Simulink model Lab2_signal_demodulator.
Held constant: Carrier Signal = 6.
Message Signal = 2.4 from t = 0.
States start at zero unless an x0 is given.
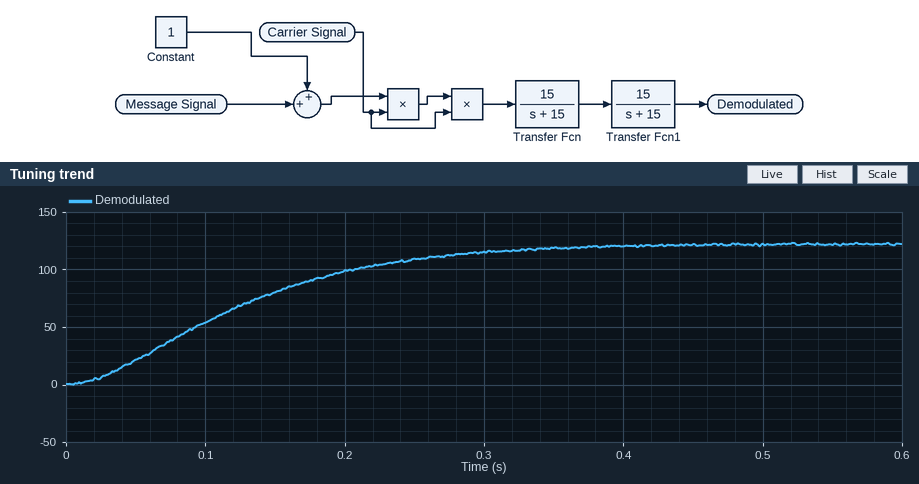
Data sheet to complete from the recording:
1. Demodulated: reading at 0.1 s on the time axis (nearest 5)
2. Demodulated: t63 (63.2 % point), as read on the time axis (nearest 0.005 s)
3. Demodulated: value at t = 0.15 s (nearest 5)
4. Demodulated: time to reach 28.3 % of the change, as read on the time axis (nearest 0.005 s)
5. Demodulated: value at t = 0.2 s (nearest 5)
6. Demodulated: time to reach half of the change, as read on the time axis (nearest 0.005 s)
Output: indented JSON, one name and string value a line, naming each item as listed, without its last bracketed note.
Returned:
{
  "Demodulated: reading at 0.1 s on the time axis": "55",
  "Demodulated: t63 (63.2 % point), as read on the time axis": "0.145 s",
  "Demodulated: value at t = 0.15 s": "80",
  "Demodulated: time to reach 28.3 % of the change, as read on the time axis": "0.070 s",
  "Demodulated: value at t = 0.2 s": "100",
  "Demodulated: time to reach half of the change, as read on the time axis": "0.110 s"
}
